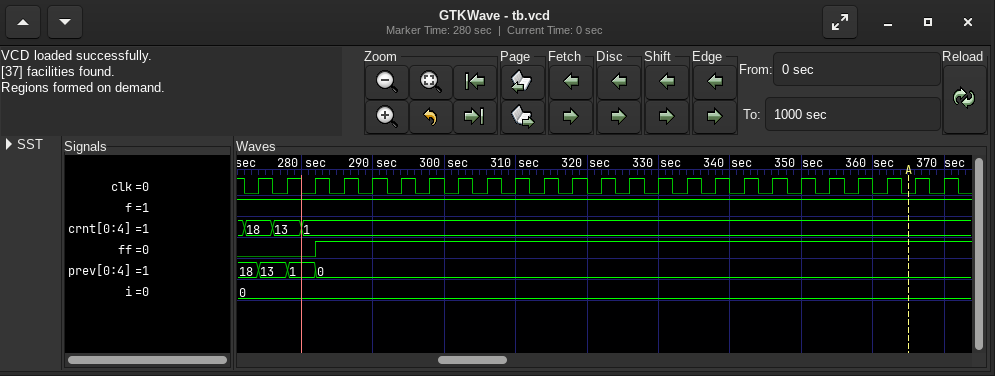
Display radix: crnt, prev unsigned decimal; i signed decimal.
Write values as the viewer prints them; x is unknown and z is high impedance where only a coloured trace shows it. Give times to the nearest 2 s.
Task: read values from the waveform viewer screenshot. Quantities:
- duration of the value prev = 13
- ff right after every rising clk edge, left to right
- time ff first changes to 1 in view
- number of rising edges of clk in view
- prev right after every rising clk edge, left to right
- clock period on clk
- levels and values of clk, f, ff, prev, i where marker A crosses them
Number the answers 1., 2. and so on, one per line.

1. 4 s
2. 0 0 1 1 1 1 1 1 1 1 1 1 1 1 1 1 1 1 1 1 1 1 1 1 1
3. 282 s
4. 25
5. 13, 1, 0, 0, 0, 0, 0, 0, 0, 0, 0, 0, 0, 0, 0, 0, 0, 0, 0, 0, 0, 0, 0, 0, 0
6. 4 s
7. clk=0, f=1, ff=1, prev=0, i=0
